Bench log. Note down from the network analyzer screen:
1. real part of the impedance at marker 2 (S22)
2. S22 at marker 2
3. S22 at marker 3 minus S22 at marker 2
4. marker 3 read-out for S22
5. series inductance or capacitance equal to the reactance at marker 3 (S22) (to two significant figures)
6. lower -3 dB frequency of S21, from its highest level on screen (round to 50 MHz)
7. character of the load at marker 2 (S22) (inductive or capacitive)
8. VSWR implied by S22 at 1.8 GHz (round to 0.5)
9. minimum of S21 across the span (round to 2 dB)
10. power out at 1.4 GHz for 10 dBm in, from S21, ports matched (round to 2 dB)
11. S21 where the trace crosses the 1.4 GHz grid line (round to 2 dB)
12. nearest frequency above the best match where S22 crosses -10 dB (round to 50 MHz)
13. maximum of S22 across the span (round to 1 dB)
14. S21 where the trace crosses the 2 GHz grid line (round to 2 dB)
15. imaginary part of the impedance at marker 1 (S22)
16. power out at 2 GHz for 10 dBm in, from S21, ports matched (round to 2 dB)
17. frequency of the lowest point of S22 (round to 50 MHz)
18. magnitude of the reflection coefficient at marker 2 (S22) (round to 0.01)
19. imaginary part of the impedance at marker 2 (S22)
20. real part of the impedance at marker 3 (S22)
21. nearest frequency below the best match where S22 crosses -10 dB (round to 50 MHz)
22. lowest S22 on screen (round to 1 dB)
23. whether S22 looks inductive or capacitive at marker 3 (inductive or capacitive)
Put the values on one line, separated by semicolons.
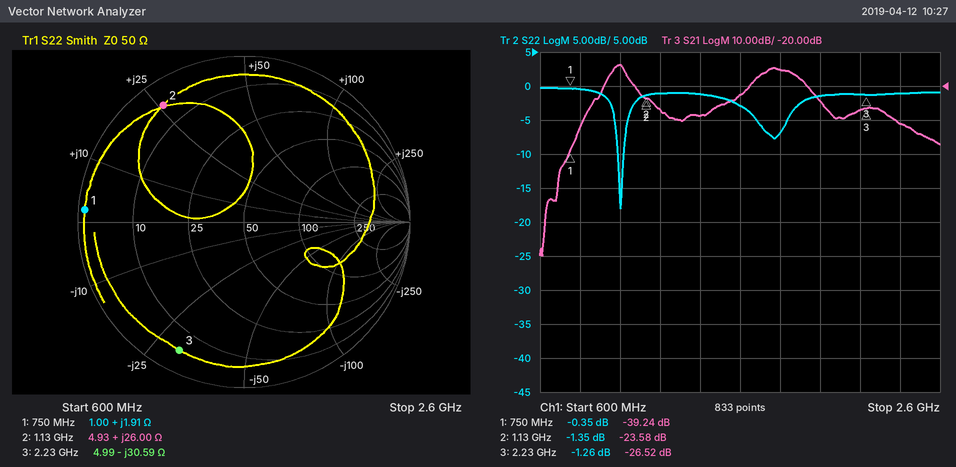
4.93 Ω; -1.35 dB; 0.09 dB; -1.26 dB; 2.3 pF; 950 MHz; inductive; 2.5; -70 dB; -18 dBm; -28 dB; 1.00 GHz; 0 dB; -24 dB; +1.91 Ω; -14 dBm; 1.00 GHz; 0.86; +26.00 Ω; 4.99 Ω; 1.00 GHz; -18 dB; capacitive
